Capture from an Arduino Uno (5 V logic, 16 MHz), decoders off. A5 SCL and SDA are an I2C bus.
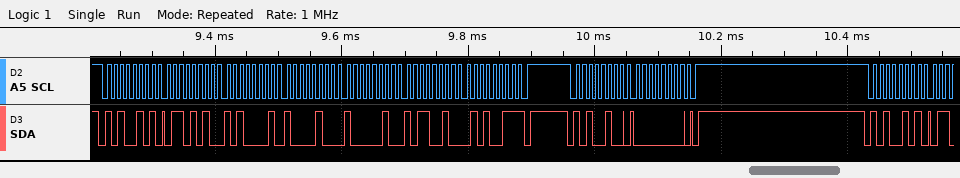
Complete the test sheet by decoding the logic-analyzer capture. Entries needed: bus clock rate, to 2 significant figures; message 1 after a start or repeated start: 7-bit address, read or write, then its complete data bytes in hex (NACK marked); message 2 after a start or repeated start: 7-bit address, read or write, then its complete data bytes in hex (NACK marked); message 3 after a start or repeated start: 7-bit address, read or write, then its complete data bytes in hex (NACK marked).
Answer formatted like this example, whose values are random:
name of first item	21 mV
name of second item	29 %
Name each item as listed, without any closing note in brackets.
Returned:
bus clock rate, to 2 significant figures	100 kHz
message 1 after a start or repeated start: 7-bit address, read or write, then its complete data bytes in hex	0x52 read: 6A A1 84 82 B2 53 NACK
message 2 after a start or repeated start: 7-bit address, read or write, then its complete data bytes in hex	0x52 write: 00
message 3 after a start or repeated start: 7-bit address, read or write, then its complete data bytes in hex	0x52 read
